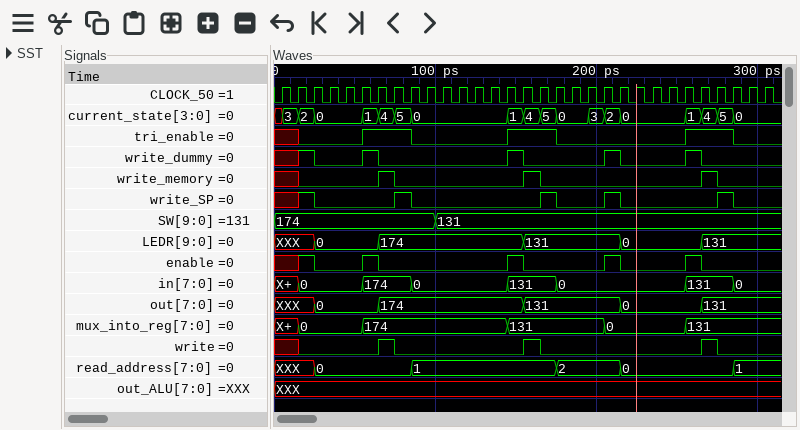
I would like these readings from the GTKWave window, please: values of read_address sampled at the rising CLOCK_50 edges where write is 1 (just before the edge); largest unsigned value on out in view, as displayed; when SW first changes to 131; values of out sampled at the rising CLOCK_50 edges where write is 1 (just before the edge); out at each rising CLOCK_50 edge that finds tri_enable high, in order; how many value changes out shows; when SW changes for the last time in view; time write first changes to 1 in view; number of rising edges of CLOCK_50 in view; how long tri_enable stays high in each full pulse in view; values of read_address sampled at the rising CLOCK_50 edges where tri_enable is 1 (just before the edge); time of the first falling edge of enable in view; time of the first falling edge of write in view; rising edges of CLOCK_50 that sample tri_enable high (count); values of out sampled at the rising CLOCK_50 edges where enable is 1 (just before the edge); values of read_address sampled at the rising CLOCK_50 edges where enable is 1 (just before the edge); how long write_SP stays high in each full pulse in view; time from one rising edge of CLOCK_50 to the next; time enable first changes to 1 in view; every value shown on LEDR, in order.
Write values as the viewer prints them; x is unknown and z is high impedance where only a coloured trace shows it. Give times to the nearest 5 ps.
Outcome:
0, 1, 0
174
100 ps
174, 131, 131
0, 174, 174, 174, 131, 131, 0, 131, 131
5
100 ps
65 ps
31
30 ps, 30 ps, 30 ps
0, 0, 0, 1, 1, 1, 0, 0, 0
25 ps
75 ps
9
XXX, 0, 174, 131, 0
XXX, 0, 1, 2, 0
10 ps, 10 ps, 10 ps, 10 ps
10 ps
15 ps
XXX, 0, 174, 131, 0, 131
